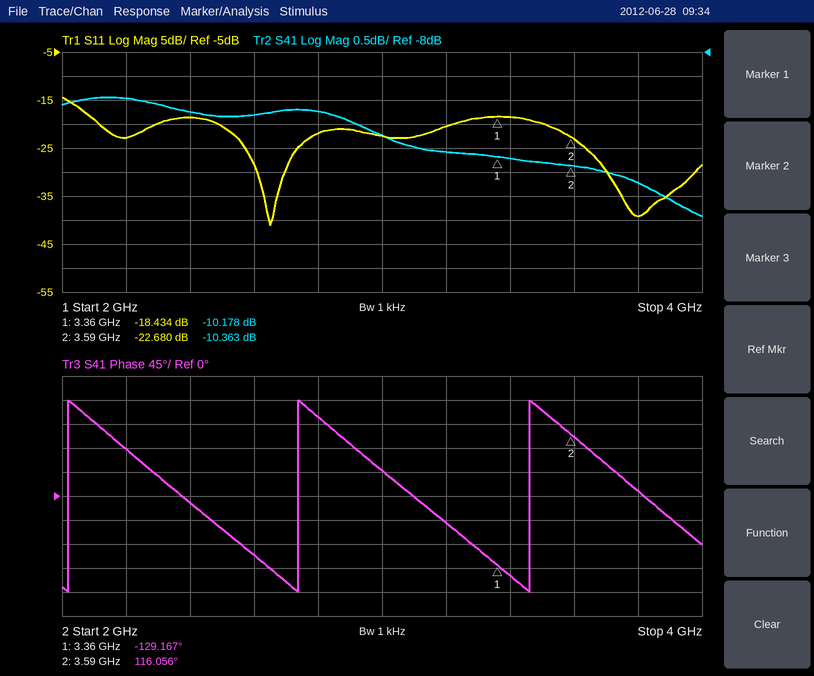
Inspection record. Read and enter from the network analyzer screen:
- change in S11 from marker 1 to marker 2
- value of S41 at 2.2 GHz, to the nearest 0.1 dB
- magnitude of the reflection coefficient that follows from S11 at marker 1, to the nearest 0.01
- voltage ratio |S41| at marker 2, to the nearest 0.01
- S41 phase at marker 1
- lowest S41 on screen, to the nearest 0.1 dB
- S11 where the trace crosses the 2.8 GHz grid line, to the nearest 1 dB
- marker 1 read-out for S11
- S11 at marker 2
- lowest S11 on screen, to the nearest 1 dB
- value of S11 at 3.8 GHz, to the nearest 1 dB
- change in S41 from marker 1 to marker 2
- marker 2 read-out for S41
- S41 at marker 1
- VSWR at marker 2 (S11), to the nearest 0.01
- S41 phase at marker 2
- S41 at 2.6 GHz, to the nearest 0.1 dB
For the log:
-4.246 dB
-9.0 dB
0.12
0.30
-129.167°
-11.4 dB
-22 dB
-18.434 dB
-22.680 dB
-41 dB
-39 dB
-0.185 dB
-10.363 dB
-10.178 dB
1.16
116.056°
-9.3 dB
